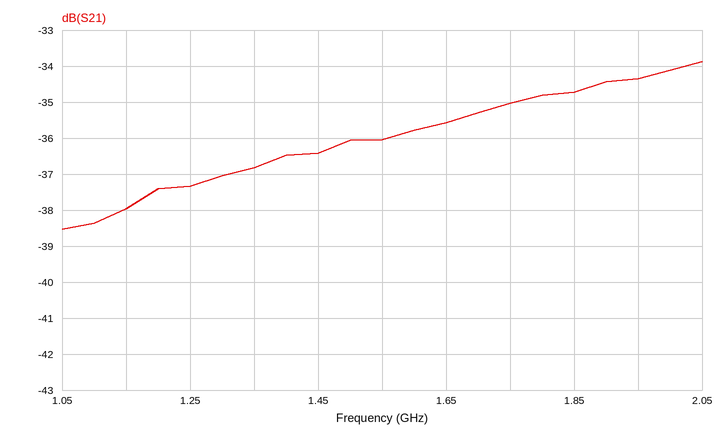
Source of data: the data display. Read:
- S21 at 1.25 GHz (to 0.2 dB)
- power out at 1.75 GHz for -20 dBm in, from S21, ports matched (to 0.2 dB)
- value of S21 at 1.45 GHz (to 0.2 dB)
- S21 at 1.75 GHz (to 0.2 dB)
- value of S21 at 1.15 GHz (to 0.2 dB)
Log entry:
-37.4 dB
-55.0 dBm
-36.4 dB
-35.0 dB
-38.0 dB
